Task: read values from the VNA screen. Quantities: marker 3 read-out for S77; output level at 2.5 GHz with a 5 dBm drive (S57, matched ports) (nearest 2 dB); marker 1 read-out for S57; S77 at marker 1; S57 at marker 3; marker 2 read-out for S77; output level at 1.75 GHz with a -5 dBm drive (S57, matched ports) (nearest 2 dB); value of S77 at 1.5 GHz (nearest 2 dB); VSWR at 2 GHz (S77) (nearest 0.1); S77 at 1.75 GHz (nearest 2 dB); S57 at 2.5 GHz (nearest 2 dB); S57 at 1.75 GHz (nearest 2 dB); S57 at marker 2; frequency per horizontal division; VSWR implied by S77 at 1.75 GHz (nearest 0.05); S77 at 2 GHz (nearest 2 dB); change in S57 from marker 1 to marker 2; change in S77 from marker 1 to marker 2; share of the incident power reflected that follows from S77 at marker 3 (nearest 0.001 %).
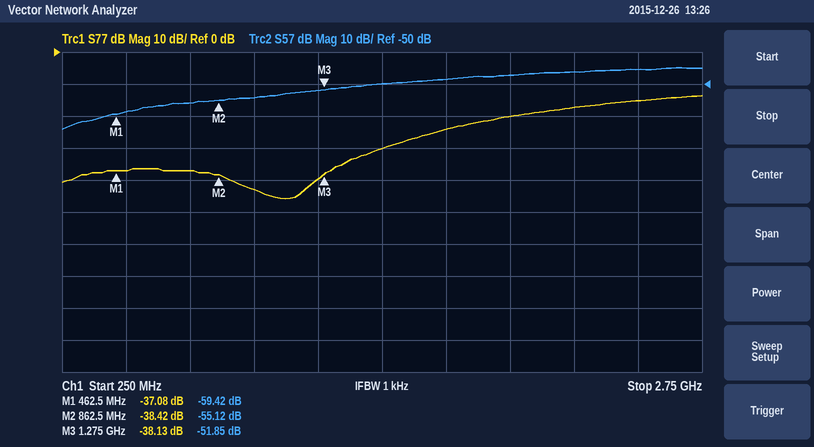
-38.13 dB
-40 dBm
-59.42 dB
-37.08 dB
-51.85 dB
-38.42 dB
-54 dBm
-30 dB
1.2
-24 dB
-46 dB
-48 dB
-55.12 dB
250 MHz
1.15
-20 dB
4.30 dB
-1.34 dB
0.015 %
